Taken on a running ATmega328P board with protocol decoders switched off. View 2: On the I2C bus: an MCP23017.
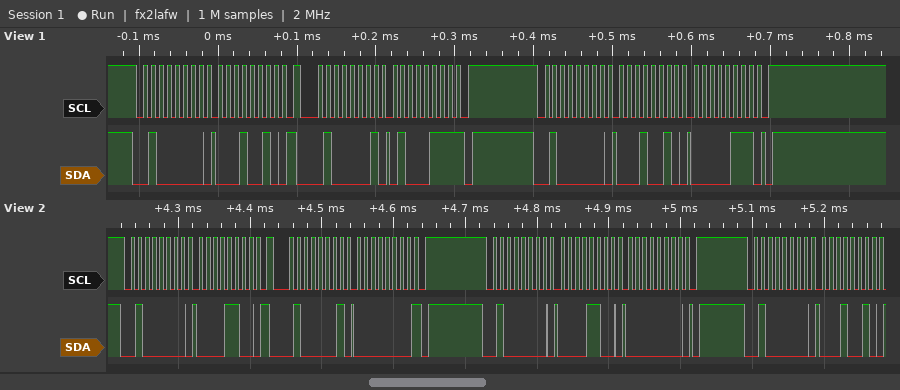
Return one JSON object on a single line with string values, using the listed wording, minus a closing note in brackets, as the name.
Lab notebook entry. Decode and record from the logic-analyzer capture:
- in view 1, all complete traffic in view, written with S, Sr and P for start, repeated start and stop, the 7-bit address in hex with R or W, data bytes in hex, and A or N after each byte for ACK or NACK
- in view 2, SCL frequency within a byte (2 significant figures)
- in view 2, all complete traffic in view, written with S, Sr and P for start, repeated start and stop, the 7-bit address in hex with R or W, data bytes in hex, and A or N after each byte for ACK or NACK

{"in view 1, all complete traffic in view, written with S, Sr and P for start, repeated start and stop, the 7-bit address in hex with R or W, data bytes in hex, and A or N after each byte for ACK or NACK": "S 20W A 12 A Sr 20R A 47 N P S 20W A 12 A 07 A P", "in view 2, SCL frequency within a byte": "100 kHz", "in view 2, all complete traffic in view, written with S, Sr and P for start, repeated start and stop, the 7-bit address in hex with R or W, data bytes in hex, and A or N after each byte for ACK or NACK": "S 20W A 0C A Sr 20R A 00 N P S 20W A 0C A 00 A P S 20W A 12 A"}
